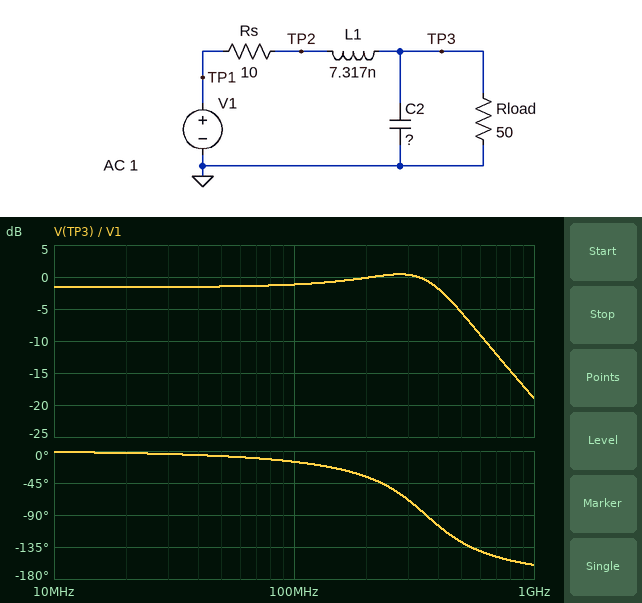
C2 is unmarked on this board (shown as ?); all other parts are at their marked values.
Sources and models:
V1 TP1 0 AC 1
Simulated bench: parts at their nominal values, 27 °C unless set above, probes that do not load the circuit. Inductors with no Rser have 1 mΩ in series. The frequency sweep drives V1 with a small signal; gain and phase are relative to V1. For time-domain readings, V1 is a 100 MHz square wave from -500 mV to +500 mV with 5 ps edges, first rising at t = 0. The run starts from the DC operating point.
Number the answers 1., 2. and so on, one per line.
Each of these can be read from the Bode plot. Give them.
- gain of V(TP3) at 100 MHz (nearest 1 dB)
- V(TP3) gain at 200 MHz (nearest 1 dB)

1. -1 dB
2. 0 dB
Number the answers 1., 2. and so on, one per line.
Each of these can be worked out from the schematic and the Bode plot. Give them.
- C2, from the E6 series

1. 33 pF
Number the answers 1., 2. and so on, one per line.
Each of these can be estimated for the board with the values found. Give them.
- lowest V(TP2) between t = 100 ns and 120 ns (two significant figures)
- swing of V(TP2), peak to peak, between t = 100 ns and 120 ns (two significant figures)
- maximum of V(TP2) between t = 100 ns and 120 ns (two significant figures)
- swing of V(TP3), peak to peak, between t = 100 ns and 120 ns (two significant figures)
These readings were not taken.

1. -580 mV
2. 1.2 V
3. 580 mV
4. 1.2 V
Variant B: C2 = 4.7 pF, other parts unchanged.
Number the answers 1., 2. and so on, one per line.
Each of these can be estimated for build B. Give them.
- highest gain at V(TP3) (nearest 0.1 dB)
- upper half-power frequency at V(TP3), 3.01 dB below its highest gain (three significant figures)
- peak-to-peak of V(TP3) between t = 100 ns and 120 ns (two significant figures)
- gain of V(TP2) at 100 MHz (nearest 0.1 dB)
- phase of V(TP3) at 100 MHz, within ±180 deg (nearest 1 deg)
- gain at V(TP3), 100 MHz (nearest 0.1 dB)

1. 0 dB
2. 1.11 GHz
3. 1.1 V
4. -1.6 dB
5. -6 deg
6. -1.5 dB
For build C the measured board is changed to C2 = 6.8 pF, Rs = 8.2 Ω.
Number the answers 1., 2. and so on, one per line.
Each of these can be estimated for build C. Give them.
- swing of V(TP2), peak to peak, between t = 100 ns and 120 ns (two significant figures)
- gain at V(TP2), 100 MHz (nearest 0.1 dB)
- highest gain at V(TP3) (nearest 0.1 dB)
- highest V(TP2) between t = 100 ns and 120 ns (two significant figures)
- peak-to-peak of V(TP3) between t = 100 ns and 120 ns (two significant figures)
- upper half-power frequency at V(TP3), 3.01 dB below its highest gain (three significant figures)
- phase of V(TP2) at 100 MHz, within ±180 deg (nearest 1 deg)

1. 1.1 V
2. -1.4 dB
3. 1.0 dB
4. 570 mV
5. 1.3 V
6. 914 MHz
7. -1 deg
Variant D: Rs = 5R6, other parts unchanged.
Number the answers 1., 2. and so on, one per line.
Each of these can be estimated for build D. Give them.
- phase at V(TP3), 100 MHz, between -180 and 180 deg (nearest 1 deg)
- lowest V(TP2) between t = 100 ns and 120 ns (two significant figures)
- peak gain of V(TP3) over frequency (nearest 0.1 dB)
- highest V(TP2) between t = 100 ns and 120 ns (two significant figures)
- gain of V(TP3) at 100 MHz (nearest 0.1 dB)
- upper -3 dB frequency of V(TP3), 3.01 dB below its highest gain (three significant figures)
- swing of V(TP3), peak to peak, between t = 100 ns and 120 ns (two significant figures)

1. -12 deg
2. -540 mV
3. 3.4 dB
4. 540 mV
5. -0.3 dB
6. 404 MHz
7. 1.5 V
